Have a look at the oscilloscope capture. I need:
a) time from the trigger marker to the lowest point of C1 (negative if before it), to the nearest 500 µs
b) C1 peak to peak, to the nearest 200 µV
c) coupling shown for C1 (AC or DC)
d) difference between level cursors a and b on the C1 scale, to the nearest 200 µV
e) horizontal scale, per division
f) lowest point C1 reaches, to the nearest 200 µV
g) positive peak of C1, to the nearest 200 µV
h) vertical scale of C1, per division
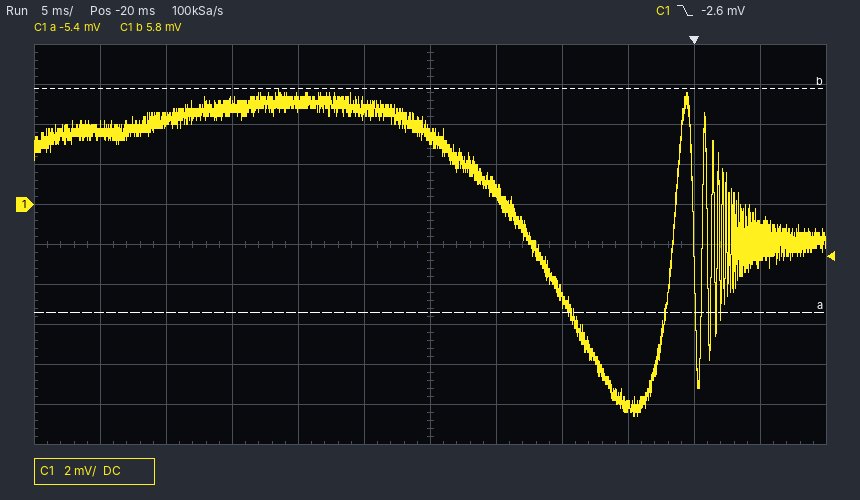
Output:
-4.5 ms
16.4 mV
DC
11.2 mV
5 ms
-10.6 mV
5.8 mV
2 mV
